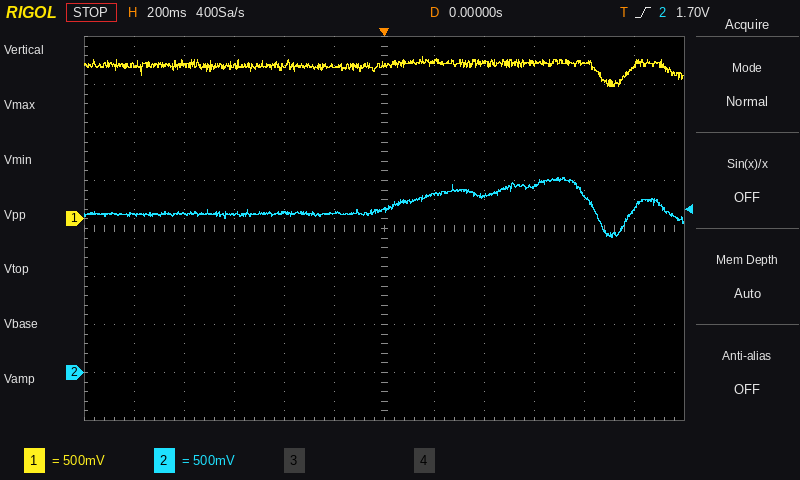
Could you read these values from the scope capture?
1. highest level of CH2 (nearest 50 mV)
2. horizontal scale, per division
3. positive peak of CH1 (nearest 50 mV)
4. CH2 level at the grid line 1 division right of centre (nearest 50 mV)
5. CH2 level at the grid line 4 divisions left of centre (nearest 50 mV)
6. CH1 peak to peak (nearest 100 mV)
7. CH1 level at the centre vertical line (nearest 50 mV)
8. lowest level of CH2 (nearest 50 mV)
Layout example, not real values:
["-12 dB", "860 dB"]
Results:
["2.05 V", "200 ms", "1.70 V", "1.85 V", "1.65 V", "300 mV", "1.60 V", "1.40 V"]
